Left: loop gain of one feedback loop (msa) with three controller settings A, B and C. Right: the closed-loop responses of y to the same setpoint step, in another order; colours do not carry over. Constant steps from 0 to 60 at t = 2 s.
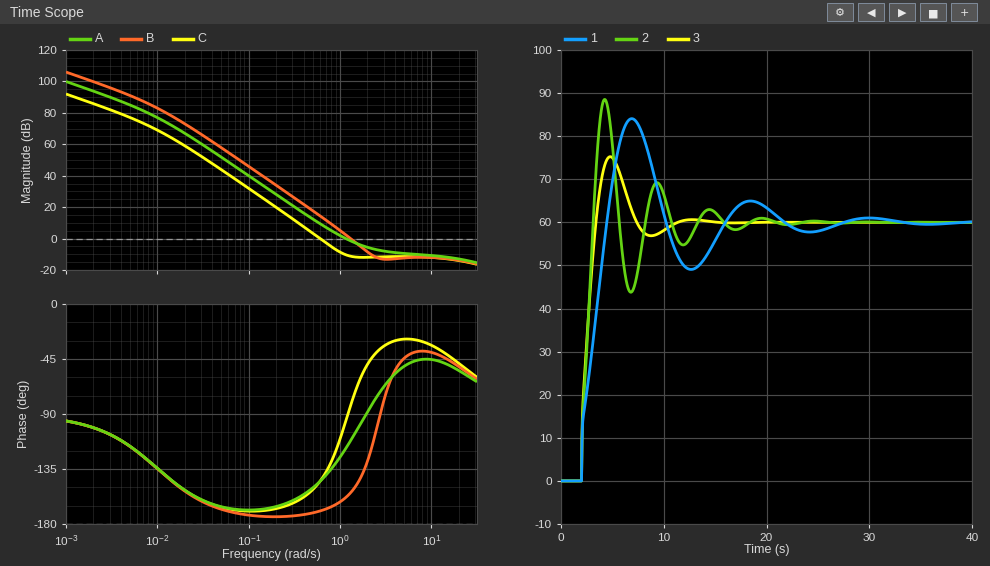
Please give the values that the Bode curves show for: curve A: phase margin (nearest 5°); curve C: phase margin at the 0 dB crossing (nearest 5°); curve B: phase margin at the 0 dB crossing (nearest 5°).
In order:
60°
35°
25°
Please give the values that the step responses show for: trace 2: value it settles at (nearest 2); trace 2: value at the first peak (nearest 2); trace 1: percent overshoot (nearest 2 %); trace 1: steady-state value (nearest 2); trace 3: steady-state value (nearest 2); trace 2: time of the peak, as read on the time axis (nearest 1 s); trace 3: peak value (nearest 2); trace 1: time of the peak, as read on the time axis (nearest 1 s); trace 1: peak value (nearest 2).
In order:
60
88
40 %
60
60
4 s
76
7 s
84
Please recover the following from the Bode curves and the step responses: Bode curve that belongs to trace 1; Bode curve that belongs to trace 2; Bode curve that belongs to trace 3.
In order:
C
B
A
